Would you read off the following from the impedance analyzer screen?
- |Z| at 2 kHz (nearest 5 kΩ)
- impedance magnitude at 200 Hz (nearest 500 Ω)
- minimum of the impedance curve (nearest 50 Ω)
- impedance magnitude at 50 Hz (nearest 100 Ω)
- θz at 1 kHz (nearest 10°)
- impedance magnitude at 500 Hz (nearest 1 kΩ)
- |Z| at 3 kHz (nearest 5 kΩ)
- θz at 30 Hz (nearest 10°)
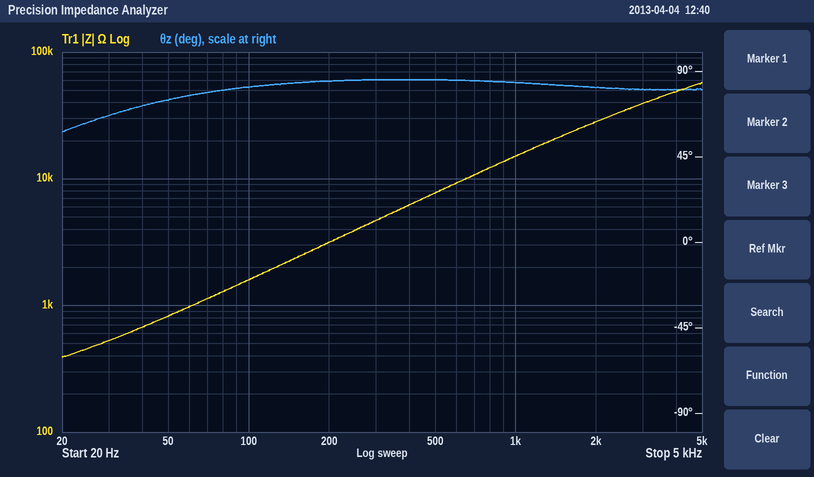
30 kΩ
3.0 kΩ
400 Ω
800 Ω
80°
8 kΩ
40 kΩ
70°
